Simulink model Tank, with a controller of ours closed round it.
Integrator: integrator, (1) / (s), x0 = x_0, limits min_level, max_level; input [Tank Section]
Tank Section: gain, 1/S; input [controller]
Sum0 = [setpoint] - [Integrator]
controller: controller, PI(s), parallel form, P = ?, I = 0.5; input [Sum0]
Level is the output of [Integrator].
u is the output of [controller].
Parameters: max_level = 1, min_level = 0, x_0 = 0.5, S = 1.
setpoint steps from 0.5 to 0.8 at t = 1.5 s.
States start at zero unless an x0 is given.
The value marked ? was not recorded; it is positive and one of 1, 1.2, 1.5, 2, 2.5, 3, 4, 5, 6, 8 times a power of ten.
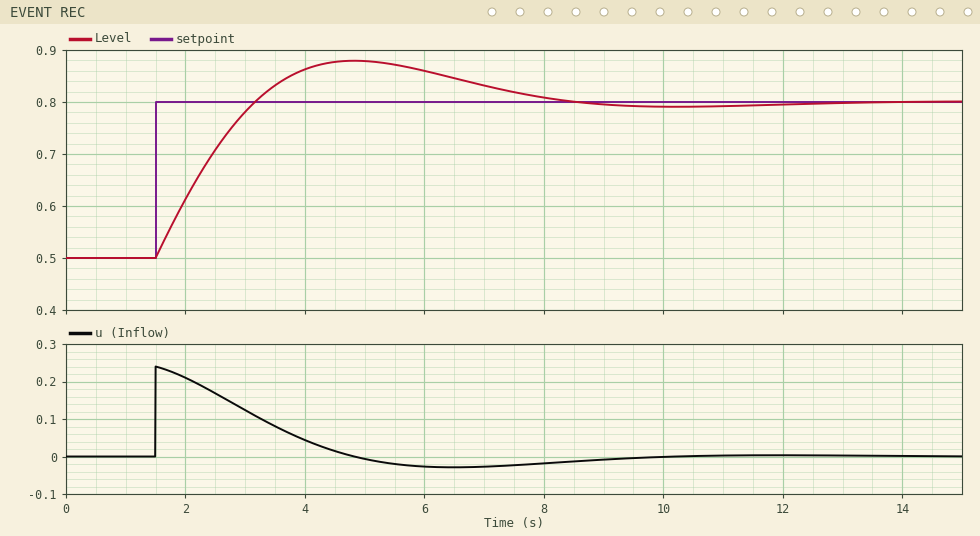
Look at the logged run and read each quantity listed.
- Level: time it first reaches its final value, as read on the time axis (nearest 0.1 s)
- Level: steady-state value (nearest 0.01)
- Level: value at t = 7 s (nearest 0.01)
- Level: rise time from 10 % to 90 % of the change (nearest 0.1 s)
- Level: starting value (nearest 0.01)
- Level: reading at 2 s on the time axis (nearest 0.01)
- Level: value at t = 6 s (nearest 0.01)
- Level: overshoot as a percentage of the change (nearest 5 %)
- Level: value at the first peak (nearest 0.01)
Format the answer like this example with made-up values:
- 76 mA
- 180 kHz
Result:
- 3.2 s
- 0.80
- 0.83
- 1.3 s
- 0.50
- 0.61
- 0.86
- 25 %
- 0.88
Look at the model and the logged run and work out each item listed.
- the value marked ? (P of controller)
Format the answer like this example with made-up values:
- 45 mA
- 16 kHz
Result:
- 0.8
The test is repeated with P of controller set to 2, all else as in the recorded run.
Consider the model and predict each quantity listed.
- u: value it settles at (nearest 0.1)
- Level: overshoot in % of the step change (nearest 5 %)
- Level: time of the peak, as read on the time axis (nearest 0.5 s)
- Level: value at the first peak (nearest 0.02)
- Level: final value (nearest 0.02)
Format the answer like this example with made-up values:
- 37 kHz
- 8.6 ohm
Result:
- 0.0
- 10 %
- 4.0 s
- 0.82
- 0.80
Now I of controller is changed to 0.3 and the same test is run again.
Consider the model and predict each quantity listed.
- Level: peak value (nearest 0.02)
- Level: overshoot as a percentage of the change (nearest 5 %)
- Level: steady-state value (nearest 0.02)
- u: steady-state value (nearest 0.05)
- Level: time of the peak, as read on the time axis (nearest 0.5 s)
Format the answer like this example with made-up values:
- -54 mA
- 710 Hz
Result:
- 0.86
- 20 %
- 0.80
- 0.00
- 5.5 s
